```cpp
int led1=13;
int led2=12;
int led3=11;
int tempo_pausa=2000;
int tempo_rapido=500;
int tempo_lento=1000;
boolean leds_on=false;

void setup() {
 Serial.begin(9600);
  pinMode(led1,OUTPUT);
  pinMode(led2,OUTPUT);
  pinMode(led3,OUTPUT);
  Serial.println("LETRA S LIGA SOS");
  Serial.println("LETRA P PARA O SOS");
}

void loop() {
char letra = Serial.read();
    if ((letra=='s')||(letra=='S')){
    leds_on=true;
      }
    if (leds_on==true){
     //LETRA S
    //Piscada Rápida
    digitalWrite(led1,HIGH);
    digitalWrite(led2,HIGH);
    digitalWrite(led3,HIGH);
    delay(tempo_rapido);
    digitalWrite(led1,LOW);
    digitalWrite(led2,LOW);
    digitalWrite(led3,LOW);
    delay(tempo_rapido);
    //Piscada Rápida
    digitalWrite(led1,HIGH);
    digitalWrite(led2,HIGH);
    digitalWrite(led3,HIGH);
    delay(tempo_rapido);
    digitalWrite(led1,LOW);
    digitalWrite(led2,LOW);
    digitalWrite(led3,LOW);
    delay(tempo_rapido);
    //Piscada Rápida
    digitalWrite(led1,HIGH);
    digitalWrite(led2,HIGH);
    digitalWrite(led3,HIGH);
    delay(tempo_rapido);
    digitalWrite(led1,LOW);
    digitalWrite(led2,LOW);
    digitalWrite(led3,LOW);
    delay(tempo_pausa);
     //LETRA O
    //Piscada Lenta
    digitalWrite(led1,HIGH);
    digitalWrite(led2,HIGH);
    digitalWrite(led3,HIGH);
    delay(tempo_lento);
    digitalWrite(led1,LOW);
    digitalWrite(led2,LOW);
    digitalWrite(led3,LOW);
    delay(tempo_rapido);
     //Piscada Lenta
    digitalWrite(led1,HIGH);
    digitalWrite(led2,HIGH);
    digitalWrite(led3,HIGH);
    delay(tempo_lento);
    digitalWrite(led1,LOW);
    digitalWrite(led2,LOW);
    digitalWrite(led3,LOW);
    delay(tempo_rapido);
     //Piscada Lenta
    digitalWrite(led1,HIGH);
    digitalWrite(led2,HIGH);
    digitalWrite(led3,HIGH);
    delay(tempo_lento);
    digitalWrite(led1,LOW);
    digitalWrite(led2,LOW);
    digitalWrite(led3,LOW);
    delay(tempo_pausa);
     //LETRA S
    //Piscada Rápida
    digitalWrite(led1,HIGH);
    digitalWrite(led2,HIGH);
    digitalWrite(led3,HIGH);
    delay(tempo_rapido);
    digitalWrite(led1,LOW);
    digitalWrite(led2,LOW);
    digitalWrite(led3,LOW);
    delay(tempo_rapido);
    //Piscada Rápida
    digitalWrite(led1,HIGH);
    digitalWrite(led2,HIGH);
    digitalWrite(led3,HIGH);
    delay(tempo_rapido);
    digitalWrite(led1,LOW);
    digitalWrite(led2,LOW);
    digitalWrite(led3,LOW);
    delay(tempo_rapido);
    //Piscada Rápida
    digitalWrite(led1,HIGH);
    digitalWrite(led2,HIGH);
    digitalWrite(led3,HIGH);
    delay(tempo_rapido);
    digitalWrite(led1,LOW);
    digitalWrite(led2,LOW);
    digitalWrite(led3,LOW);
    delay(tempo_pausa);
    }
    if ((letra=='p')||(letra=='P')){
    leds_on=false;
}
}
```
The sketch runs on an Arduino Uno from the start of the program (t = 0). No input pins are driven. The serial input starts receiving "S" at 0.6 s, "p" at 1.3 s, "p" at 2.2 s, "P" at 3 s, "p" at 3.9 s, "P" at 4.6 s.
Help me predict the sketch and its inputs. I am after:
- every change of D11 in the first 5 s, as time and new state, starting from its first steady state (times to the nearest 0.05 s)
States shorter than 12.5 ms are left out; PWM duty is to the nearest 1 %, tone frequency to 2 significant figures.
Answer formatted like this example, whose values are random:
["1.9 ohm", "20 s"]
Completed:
["0 s low; 0.6 s high; 1.1 s low; 1.6 s high; 2.1 s low; 2.6 s high; 3.1 s low"]
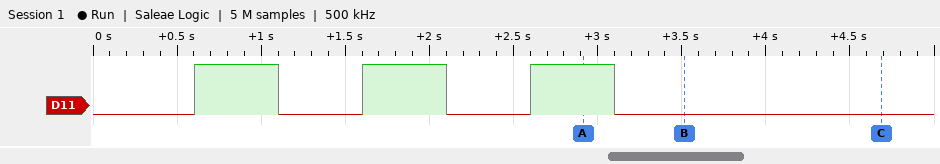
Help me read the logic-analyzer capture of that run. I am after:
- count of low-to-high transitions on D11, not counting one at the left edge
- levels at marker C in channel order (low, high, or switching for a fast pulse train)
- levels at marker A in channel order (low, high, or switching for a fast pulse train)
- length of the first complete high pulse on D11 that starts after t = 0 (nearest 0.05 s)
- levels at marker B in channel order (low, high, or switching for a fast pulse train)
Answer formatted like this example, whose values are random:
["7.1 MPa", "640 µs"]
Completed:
["3", "D11 low", "D11 high", "0.50 s", "D11 low"]
